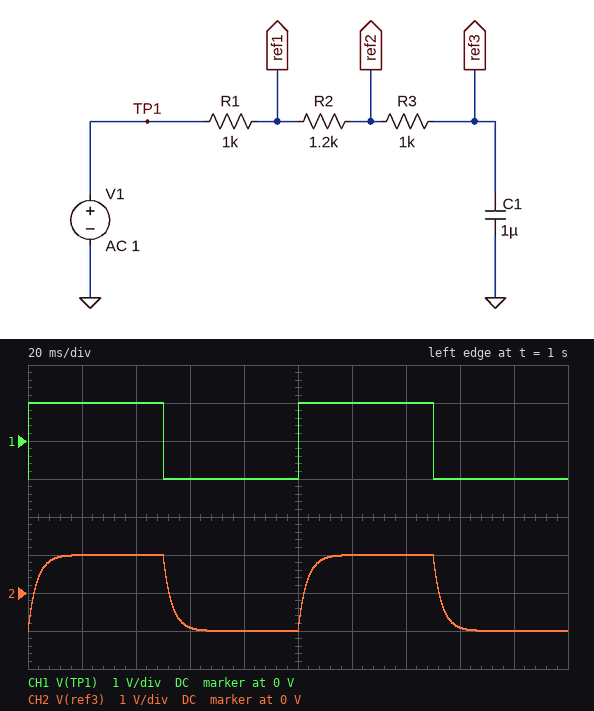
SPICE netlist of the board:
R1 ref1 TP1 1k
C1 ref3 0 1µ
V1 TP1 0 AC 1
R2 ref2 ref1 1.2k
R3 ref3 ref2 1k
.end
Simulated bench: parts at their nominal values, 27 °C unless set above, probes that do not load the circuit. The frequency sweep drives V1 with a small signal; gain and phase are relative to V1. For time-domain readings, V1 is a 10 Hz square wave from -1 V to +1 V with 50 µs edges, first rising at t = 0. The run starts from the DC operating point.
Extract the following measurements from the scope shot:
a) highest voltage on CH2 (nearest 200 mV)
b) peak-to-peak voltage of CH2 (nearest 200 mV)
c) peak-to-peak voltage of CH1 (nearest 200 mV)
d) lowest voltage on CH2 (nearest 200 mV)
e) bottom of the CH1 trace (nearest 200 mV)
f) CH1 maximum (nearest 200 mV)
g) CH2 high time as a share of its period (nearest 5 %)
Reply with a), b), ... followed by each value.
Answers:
a) 1.0 V
b) 2.0 V
c) 2.0 V
d) -1.0 V
e) -1.0 V
f) 1.0 V
g) 50 %
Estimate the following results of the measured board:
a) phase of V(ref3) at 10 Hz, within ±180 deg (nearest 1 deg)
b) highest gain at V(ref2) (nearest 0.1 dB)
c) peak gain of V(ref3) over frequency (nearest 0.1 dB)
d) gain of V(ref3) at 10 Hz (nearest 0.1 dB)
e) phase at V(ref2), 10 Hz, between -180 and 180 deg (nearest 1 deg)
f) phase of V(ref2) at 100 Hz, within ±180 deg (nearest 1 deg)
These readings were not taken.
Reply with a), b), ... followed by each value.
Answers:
a) -11 deg
b) 0 dB
c) 0 dB
d) -0.2 dB
e) -8 deg
f) -31 deg
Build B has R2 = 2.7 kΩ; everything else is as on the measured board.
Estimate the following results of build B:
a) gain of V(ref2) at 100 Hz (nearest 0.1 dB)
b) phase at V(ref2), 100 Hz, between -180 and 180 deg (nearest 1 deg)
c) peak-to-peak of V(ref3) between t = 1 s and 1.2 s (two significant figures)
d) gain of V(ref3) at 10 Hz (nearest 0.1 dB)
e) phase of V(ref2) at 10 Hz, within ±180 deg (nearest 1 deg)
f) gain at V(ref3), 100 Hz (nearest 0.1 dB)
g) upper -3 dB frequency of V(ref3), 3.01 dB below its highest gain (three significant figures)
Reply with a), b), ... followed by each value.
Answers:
a) -8.4 dB
b) -39 deg
c) 2.0 V
d) -0.4 dB
e) -13 deg
f) -9.9 dB
g) 33.9 Hz
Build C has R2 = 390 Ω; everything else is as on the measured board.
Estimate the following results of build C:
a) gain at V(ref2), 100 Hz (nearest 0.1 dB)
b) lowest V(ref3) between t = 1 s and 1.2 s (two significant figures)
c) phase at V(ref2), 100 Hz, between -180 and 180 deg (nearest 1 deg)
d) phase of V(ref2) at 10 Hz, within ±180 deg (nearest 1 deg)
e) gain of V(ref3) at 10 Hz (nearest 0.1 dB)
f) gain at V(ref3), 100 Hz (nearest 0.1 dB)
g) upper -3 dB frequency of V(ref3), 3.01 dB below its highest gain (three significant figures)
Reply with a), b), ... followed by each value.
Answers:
a) -3.7 dB
b) -1.0 V
c) -24 deg
d) -5 deg
e) -0.1 dB
f) -5.1 dB
g) 66.6 Hz
